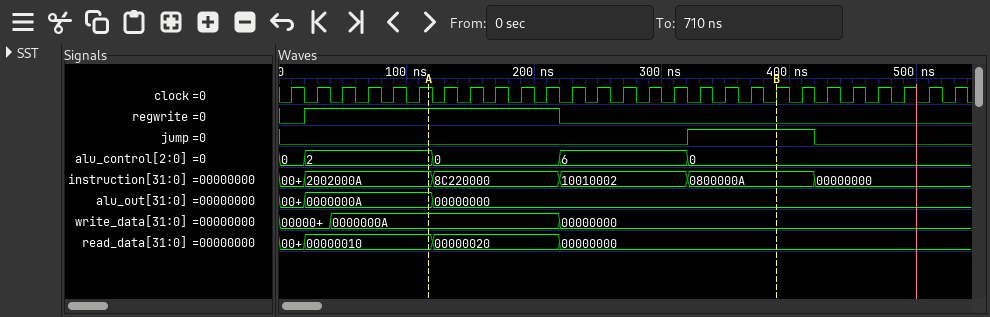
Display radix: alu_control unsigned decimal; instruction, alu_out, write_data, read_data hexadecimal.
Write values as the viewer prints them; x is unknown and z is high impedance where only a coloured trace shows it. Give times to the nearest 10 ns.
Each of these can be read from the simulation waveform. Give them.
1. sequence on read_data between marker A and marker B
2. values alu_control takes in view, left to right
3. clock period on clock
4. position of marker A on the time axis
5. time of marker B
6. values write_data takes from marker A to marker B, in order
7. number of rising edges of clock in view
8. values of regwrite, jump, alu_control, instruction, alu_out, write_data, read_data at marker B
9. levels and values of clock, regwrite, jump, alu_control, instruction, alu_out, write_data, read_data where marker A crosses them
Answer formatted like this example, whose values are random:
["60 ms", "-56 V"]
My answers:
["00000010, 00000020, 00000000", "0, 2, 0, 6, 0", "20 ns", "120 ns", "390 ns", "0000000A, 00000000", "27", "regwrite=0, jump=1, alu_control=0, instruction=0800000A, alu_out=00000000, write_data=00000000, read_data=00000000", "clock=1, regwrite=1, jump=0, alu_control=2, instruction=2002000A, alu_out=0000000A, write_data=0000000A, read_data=00000010"]
